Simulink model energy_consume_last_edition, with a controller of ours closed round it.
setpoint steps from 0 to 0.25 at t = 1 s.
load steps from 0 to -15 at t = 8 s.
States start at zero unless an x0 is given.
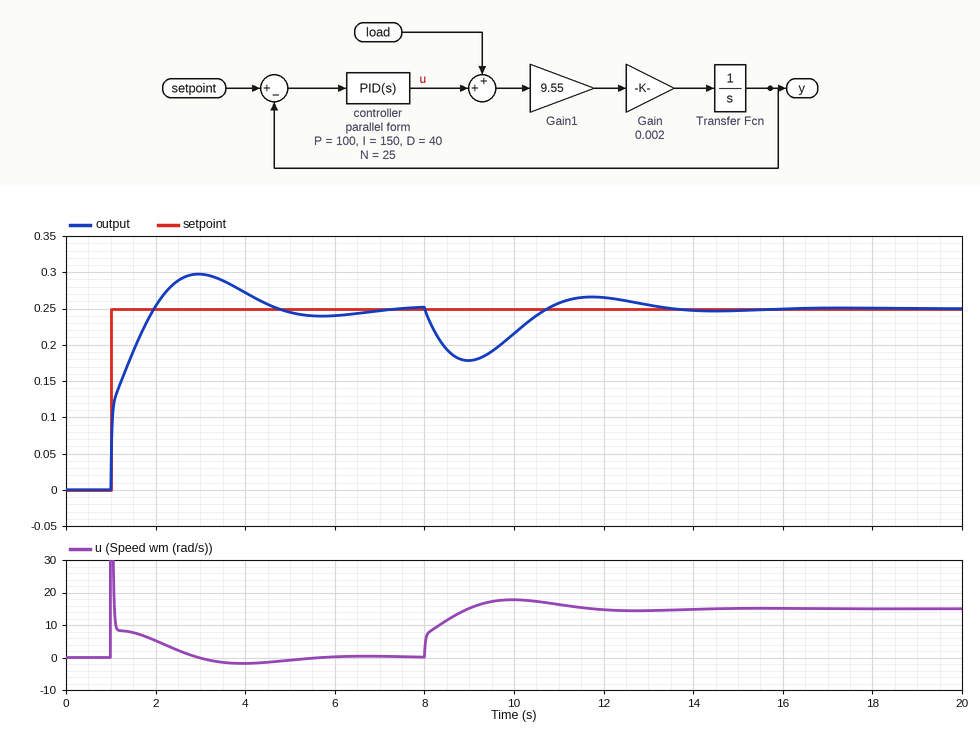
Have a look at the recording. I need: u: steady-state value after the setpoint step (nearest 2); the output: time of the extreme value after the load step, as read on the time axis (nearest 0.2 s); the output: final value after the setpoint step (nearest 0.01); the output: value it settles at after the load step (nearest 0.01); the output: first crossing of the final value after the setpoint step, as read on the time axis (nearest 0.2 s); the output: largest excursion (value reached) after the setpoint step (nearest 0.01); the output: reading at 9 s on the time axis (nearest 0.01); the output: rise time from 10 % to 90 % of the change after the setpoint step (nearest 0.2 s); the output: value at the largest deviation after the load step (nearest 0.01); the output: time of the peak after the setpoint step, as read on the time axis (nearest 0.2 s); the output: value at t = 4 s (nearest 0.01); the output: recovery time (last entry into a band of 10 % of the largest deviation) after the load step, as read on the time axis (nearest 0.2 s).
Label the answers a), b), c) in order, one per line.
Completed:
a) 0
b) 9.0 s
c) 0.25
d) 0.25
e) 2.0 s
f) 0.30
g) 0.18
h) 0.8 s
i) 0.18
j) 3.0 s
k) 0.27
l) 12.8 s
